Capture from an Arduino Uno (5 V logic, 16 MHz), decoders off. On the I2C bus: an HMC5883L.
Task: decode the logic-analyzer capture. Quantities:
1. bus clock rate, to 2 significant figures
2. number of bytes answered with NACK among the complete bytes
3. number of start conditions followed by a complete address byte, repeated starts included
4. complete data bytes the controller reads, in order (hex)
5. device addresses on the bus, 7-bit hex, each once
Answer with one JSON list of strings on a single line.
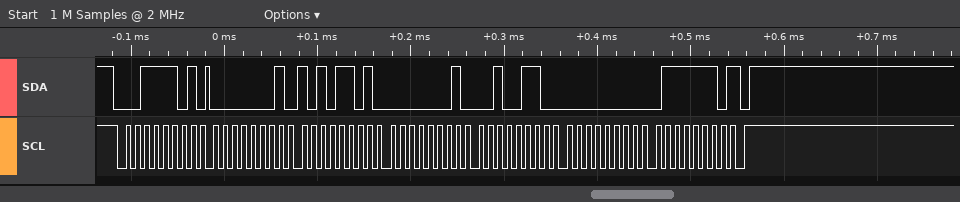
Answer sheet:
["100 kHz", "1", "1", "01 AD 01 26 00 7E", "0x1E"]
